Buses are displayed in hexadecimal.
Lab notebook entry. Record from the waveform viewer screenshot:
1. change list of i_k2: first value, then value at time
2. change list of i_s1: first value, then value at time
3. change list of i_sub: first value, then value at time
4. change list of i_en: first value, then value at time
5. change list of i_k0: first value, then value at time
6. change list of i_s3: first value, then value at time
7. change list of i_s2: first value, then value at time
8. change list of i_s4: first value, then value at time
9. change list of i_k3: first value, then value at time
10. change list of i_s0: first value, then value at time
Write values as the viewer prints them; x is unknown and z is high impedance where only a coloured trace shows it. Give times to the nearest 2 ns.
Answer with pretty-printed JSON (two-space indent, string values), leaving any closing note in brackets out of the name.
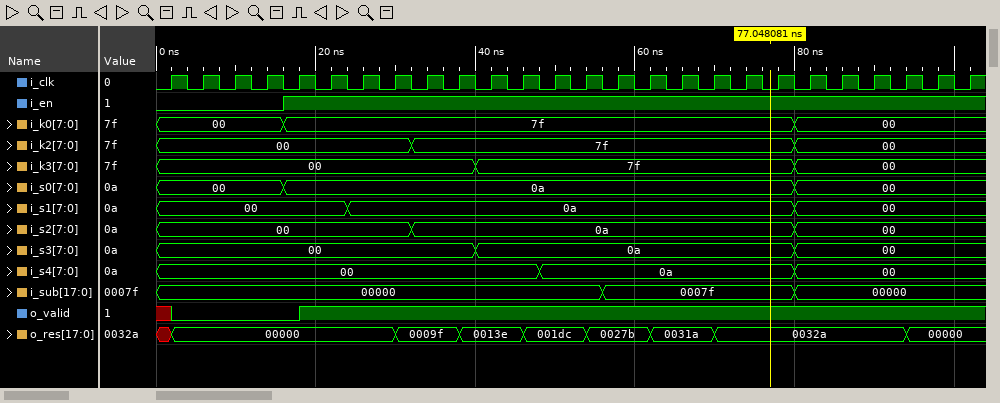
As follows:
{
  "change list of i_k2: first value, then value at time": "00, 7f at 32 ns, 00 at 80 ns",
  "change list of i_s1: first value, then value at time": "00, 0a at 24 ns, 00 at 80 ns",
  "change list of i_sub: first value, then value at time": "00000, 0007f at 56 ns, 00000 at 80 ns",
  "change list of i_en: first value, then value at time": "0, 1 at 16 ns",
  "change list of i_k0: first value, then value at time": "00, 7f at 16 ns, 00 at 80 ns",
  "change list of i_s3: first value, then value at time": "00, 0a at 40 ns, 00 at 80 ns",
  "change list of i_s2: first value, then value at time": "00, 0a at 32 ns, 00 at 80 ns",
  "change list of i_s4: first value, then value at time": "00, 0a at 48 ns, 00 at 80 ns",
  "change list of i_k3: first value, then value at time": "00, 7f at 40 ns, 00 at 80 ns",
  "change list of i_s0: first value, then value at time": "00, 0a at 16 ns, 00 at 80 ns"
}
